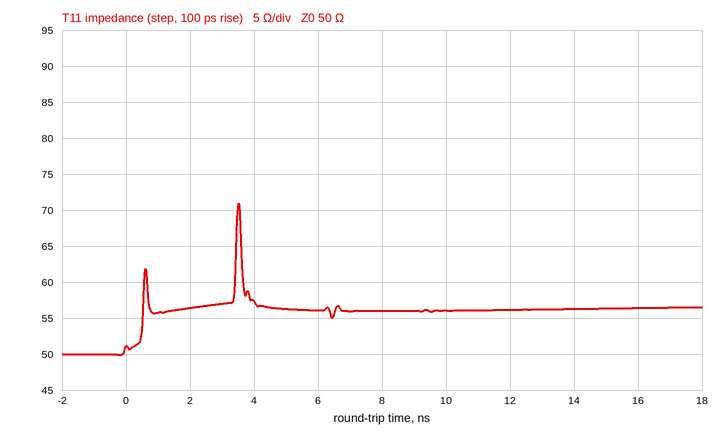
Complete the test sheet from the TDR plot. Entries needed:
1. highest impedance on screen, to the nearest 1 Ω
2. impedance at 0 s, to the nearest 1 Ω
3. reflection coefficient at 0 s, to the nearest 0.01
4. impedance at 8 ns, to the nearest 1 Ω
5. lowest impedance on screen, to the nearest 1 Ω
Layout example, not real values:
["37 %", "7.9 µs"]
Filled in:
["71 Ω", "51 Ω", "+0.01", "56 Ω", "50 Ω"]
